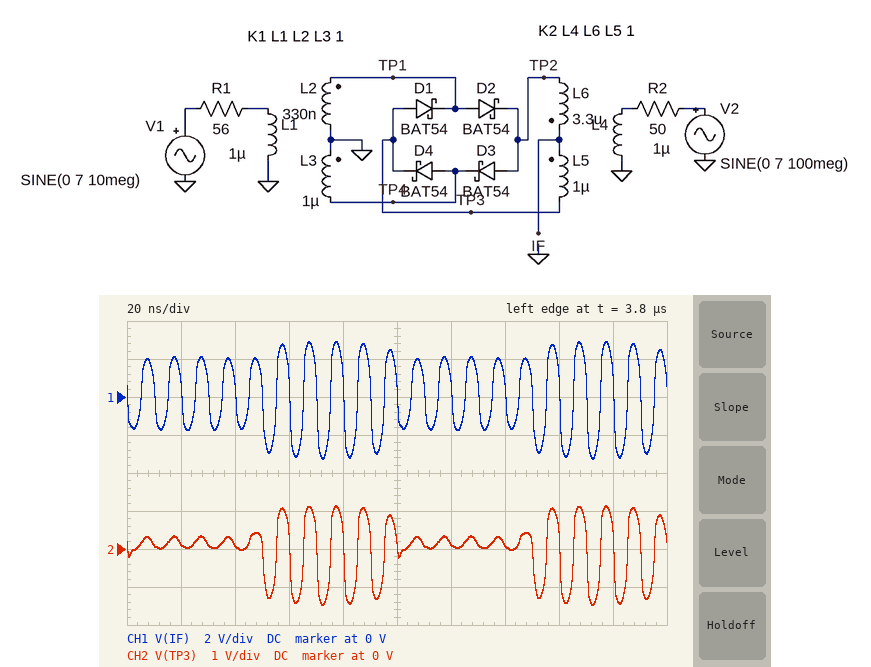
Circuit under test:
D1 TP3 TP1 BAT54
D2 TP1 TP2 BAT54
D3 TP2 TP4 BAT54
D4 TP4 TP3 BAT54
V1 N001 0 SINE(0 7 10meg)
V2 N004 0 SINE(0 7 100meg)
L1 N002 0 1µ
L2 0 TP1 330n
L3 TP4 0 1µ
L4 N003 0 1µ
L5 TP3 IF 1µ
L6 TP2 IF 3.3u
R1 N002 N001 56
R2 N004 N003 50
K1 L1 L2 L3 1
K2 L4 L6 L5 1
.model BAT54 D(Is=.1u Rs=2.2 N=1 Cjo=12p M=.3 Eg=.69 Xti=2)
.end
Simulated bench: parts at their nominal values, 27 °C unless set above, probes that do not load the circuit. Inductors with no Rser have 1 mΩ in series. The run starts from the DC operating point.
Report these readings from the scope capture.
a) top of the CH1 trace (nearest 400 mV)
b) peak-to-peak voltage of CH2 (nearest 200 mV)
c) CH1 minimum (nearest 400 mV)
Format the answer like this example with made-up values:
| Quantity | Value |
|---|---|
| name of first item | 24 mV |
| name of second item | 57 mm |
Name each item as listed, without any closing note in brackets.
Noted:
| Quantity | Value |
|---|---|
| top of the CH1 trace | 2.8 V |
| peak-to-peak voltage of CH2 | 2.6 V |
| CH1 minimum | -3.2 V |
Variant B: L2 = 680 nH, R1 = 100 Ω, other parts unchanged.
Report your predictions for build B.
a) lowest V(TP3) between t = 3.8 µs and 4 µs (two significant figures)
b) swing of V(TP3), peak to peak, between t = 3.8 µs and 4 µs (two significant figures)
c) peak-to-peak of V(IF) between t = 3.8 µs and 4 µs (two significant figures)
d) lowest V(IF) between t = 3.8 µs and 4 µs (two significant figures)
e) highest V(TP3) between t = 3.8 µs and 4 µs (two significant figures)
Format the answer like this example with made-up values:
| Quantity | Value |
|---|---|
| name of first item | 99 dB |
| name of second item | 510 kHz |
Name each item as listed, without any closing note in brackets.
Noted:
| Quantity | Value |
|---|---|
| lowest V(TP3) between t = 3.8 µs and 4 µs | -1.3 V |
| swing of V(TP3), peak to peak, between t = 3.8 µs and 4 µs | 2.4 V |
| peak-to-peak of V(IF) between t = 3.8 µs and 4 µs | 5.8 V |
| lowest V(IF) between t = 3.8 µs and 4 µs | -3.0 V |
| highest V(TP3) between t = 3.8 µs and 4 µs | 1.2 V |
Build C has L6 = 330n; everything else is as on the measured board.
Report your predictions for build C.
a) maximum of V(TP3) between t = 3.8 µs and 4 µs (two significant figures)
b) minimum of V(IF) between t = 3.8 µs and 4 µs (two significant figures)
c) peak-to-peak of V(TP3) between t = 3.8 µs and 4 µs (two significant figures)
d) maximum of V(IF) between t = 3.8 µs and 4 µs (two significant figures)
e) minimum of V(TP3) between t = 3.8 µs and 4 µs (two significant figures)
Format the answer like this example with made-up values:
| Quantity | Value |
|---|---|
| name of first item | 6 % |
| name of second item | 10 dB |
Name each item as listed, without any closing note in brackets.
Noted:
| Quantity | Value |
|---|---|
| maximum of V(TP3) between t = 3.8 µs and 4 µs | 1.2 V |
| minimum of V(IF) between t = 3.8 µs and 4 µs | -3.3 V |
| peak-to-peak of V(TP3) between t = 3.8 µs and 4 µs | 2.8 V |
| maximum of V(IF) between t = 3.8 µs and 4 µs | 3.7 V |
| minimum of V(TP3) between t = 3.8 µs and 4 µs | -1.6 V |
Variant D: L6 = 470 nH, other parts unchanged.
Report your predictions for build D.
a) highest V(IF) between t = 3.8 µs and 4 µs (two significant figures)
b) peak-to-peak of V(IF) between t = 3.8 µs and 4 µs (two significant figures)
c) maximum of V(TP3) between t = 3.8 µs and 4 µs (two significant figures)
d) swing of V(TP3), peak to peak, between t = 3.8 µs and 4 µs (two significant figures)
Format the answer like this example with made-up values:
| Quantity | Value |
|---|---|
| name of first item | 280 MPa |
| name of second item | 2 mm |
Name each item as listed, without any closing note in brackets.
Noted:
| Quantity | Value |
|---|---|
| highest V(IF) between t = 3.8 µs and 4 µs | 4.8 V |
| peak-to-peak of V(IF) between t = 3.8 µs and 4 µs | 9.3 V |
| maximum of V(TP3) between t = 3.8 µs and 4 µs | 1.2 V |
| swing of V(TP3), peak to peak, between t = 3.8 µs and 4 µs | 2.7 V |
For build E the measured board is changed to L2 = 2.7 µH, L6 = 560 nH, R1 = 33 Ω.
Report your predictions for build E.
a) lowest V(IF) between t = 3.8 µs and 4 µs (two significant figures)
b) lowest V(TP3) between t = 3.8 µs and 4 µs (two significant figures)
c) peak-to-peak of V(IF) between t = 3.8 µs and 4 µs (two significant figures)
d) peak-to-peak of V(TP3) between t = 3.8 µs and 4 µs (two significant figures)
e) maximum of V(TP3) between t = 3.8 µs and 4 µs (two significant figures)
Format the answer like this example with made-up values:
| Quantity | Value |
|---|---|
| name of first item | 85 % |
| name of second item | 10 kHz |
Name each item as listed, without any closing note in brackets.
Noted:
| Quantity | Value |
|---|---|
| lowest V(IF) between t = 3.8 µs and 4 µs | -5.6 V |
| lowest V(TP3) between t = 3.8 µs and 4 µs | -1.1 V |
| peak-to-peak of V(IF) between t = 3.8 µs and 4 µs | 11 V |
| peak-to-peak of V(TP3) between t = 3.8 µs and 4 µs | 2.5 V |
| maximum of V(TP3) between t = 3.8 µs and 4 µs | 1.4 V |
